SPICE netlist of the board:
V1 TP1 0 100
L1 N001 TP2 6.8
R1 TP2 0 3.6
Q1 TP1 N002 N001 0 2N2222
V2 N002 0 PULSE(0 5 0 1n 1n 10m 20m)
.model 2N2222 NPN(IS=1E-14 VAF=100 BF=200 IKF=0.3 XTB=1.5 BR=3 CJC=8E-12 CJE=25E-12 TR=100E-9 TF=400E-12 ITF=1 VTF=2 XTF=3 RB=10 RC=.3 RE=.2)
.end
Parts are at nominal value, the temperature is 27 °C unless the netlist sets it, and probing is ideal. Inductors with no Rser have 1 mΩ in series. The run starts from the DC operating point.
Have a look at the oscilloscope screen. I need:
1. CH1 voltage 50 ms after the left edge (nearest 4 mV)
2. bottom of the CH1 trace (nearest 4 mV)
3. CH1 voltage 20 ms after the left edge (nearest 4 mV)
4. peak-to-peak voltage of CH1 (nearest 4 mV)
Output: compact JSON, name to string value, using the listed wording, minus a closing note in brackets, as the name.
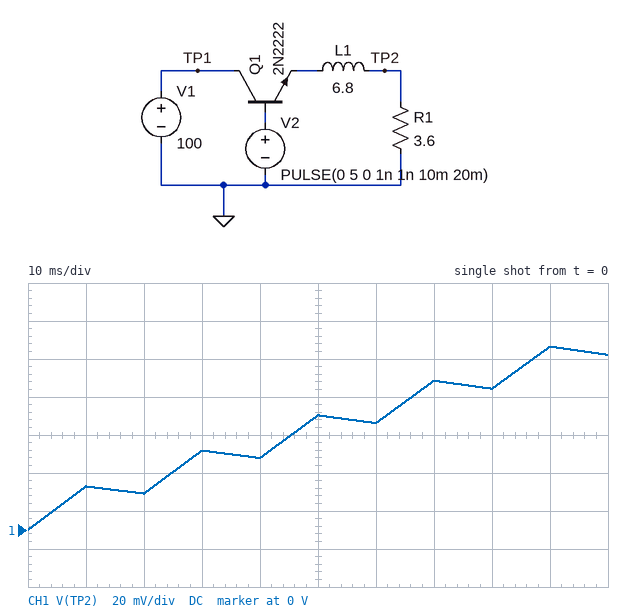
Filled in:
{"CH1 voltage 50 ms after the left edge": "60 mV", "bottom of the CH1 trace": "0 V", "CH1 voltage 20 ms after the left edge": "20 mV", "peak-to-peak voltage of CH1": "96 mV"}
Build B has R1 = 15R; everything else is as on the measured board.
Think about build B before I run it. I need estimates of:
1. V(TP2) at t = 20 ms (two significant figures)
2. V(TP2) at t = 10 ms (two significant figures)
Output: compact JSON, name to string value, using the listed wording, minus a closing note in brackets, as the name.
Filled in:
{"V(TP2) at t = 20 ms": "78 mV", "V(TP2) at t = 10 ms": "95 mV"}
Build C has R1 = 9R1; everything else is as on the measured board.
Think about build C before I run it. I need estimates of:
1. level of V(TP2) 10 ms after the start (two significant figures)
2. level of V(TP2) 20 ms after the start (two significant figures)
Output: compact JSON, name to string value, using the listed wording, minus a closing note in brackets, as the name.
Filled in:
{"level of V(TP2) 10 ms after the start": "58 mV", "level of V(TP2) 20 ms after the start": "48 mV"}
